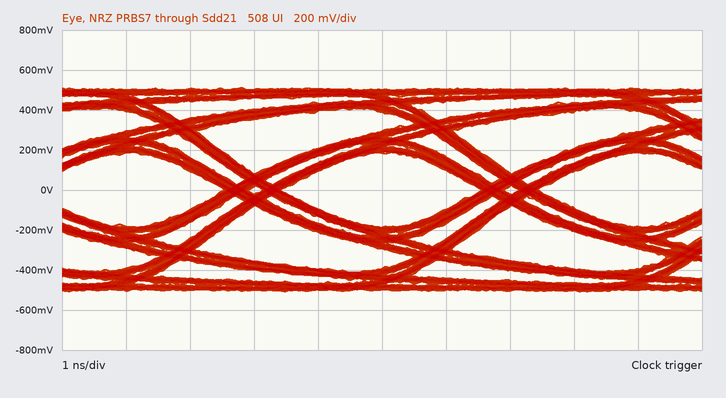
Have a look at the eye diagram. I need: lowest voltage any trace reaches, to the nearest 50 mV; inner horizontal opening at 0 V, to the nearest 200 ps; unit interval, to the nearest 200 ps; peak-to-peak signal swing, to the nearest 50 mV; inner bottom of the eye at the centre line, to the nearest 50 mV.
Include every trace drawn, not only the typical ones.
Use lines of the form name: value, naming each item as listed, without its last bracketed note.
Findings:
lowest voltage any trace reaches, to the nearest 50 mV: -500 mV
inner horizontal opening at 0 V, to the nearest 200 ps: 3.2 ns
unit interval, to the nearest 200 ps: 4.0 ns
peak-to-peak signal swing, to the nearest 50 mV: 1.00 V
inner bottom of the eye at the centre line, to the nearest 50 mV: -200 mV
